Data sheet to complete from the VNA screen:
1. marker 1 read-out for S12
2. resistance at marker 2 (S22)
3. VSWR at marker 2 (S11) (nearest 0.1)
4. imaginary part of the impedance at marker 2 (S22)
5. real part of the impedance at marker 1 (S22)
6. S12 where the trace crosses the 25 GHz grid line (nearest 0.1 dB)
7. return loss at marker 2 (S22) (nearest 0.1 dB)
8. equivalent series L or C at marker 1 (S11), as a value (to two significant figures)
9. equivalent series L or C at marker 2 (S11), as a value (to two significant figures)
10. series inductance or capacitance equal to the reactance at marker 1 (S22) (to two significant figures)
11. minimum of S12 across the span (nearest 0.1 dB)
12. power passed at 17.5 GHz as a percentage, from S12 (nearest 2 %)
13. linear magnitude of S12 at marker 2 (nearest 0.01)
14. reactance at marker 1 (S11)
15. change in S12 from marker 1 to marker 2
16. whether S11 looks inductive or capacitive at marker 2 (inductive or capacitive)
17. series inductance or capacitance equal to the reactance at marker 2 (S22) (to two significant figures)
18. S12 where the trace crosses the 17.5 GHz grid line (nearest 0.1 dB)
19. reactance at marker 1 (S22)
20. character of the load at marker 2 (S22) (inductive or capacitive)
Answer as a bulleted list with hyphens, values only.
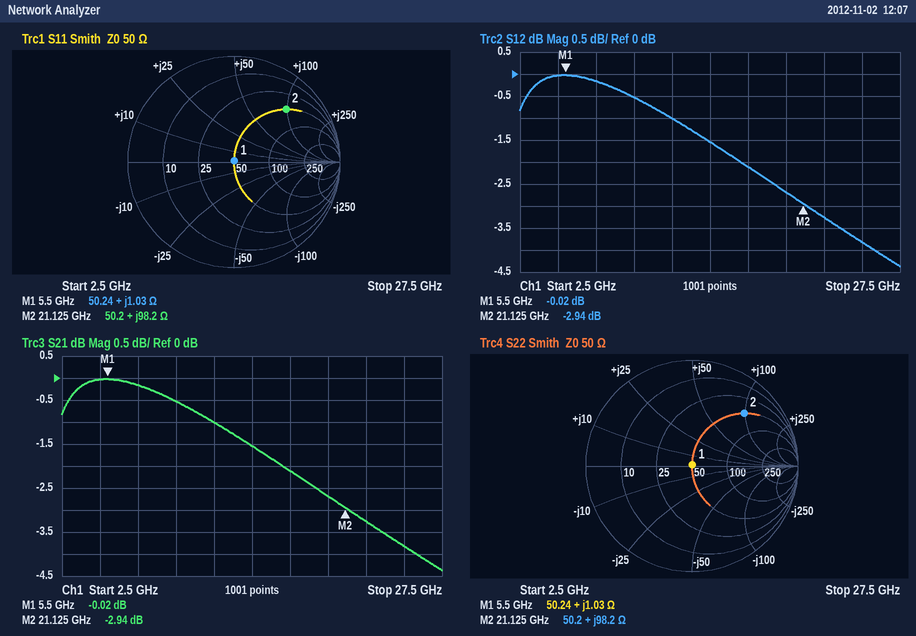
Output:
- -0.02 dB
- 50.2 Ω
- 5.7
- +98.2 Ω
- 50.24 Ω
- -3.8 dB
- 3.1 dB
- 30 pH
- 740 pH
- 30 pH
- -4.4 dB
- 62 %
- 0.71
- +1.03 Ω
- -2.92 dB
- inductive
- 740 pH
- -2.1 dB
- +1.03 Ω
- inductive
